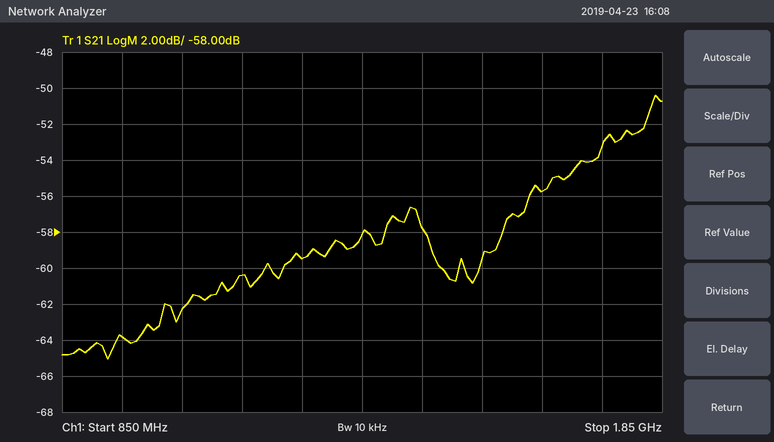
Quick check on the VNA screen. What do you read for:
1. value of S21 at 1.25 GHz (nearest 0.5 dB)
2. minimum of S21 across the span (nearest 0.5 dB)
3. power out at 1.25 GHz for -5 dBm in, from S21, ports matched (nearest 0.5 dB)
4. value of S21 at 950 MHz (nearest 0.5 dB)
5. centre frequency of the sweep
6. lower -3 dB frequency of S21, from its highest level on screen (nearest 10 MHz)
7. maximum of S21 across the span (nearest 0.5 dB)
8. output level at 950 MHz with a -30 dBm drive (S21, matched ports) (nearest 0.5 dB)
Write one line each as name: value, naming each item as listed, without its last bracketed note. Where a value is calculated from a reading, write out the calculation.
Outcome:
value of S21 at 1.25 GHz: -59.5 dB
minimum of S21 across the span: -65.0 dB
power out at 1.25 GHz for -5 dBm in, from S21, ports matched: -5 dBm + (-59.5 dB) = -64.5 dBm
value of S21 at 950 MHz: -64.0 dB
centre frequency of the sweep: 1.35 GHz
lower -3 dB frequency of S21, from its highest level on screen: 1.75 GHz
maximum of S21 across the span: -50.5 dB
output level at 950 MHz with a -30 dBm drive (S21, matched ports): -30 dBm + (-64.0 dB) = -94.0 dBm
